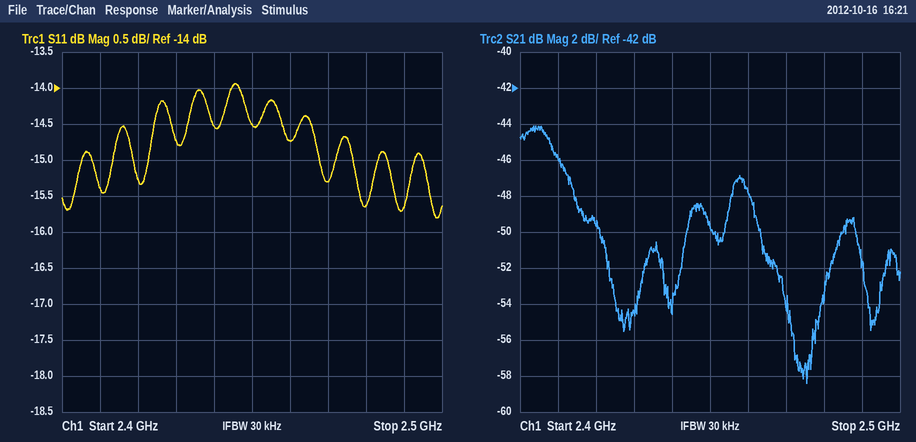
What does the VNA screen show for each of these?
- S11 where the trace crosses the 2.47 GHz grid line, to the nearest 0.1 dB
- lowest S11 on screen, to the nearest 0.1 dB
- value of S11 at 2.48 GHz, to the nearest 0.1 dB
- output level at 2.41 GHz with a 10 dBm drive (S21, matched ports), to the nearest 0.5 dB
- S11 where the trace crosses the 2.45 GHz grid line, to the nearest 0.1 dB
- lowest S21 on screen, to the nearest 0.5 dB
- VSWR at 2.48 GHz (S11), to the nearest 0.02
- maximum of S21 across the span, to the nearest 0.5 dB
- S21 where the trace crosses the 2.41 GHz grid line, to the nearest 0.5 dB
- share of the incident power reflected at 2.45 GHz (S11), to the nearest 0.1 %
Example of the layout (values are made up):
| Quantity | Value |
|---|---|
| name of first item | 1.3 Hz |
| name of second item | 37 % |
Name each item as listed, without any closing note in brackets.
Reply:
| Quantity | Value |
|---|---|
| S11 where the trace crosses the 2.47 GHz grid line, to the nearest 0.1 dB | -15.3 dB |
| lowest S11 on screen, to the nearest 0.1 dB | -15.8 dB |
| value of S11 at 2.48 GHz, to the nearest 0.1 dB | -15.6 dB |
| output level at 2.41 GHz with a 10 dBm drive (S21, matched ports), to the nearest 0.5 dB | -36.0 dBm |
| S11 where the trace crosses the 2.45 GHz grid line, to the nearest 0.1 dB | -14.5 dB |
| lowest S21 on screen, to the nearest 0.5 dB | -58.5 dB |
| VSWR at 2.48 GHz (S11), to the nearest 0.02 | 1.40 |
| maximum of S21 across the span, to the nearest 0.5 dB | -44.0 dB |
| S21 where the trace crosses the 2.41 GHz grid line, to the nearest 0.5 dB | -46.0 dB |
| share of the incident power reflected at 2.45 GHz (S11), to the nearest 0.1 % | 3.5 % |
